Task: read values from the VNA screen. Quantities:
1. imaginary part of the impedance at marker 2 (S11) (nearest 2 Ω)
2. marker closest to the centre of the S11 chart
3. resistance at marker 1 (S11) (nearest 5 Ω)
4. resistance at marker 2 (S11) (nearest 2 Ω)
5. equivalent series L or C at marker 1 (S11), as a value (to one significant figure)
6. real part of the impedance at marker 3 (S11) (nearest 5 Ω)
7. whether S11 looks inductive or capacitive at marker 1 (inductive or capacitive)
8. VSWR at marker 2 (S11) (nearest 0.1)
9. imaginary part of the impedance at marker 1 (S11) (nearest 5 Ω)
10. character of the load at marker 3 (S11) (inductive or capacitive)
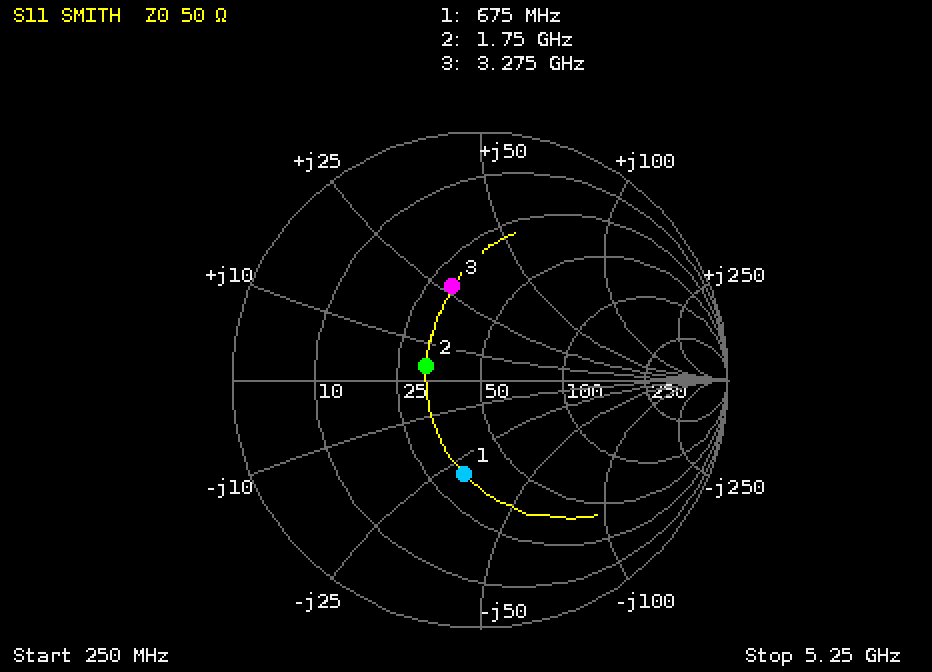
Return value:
+4 Ω
marker 2
35 Ω
32 Ω
8 pF
30 Ω
capacitive
1.6
-30 Ω
inductive
